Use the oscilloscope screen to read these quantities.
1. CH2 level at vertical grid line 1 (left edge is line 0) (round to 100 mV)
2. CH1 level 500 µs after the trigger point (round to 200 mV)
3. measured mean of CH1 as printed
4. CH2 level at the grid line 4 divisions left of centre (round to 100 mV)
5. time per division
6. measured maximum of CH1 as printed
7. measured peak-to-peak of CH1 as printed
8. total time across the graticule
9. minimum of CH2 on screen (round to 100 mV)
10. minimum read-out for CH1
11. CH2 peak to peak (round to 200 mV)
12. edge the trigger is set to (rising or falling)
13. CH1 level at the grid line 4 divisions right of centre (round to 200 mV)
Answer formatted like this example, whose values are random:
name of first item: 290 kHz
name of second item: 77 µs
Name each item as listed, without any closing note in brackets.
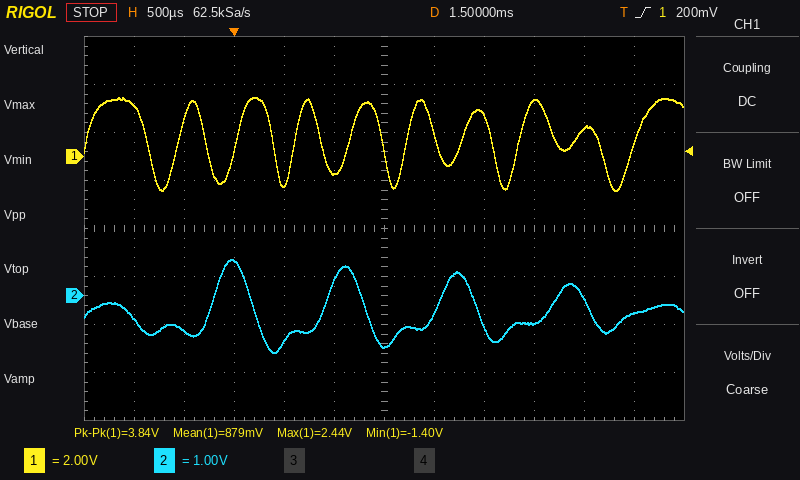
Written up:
CH2 level at vertical grid line 1 (left edge is line 0): -500 mV
CH1 level 500 µs after the trigger point: -1.2 V
measured mean of CH1 as printed: 879 mV
CH2 level at the grid line 4 divisions left of centre: -700 mV
time per division: 500 µs
measured maximum of CH1 as printed: 2.44 V
measured peak-to-peak of CH1 as printed: 3.84 V
total time across the graticule: 6 ms
minimum of CH2 on screen: -1.2 V
minimum read-out for CH1: -1.40 V
CH2 peak to peak: 2.0 V
edge the trigger is set to: rising
CH1 level at the grid line 4 divisions right of centre: 1.2 V
